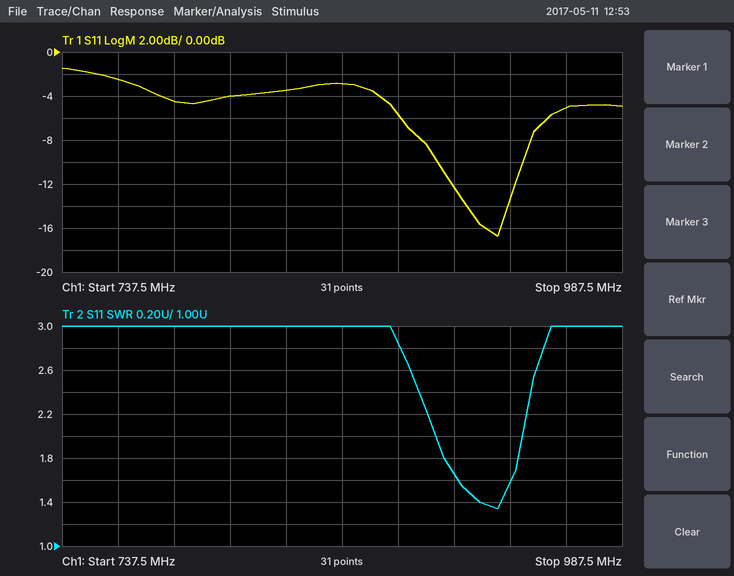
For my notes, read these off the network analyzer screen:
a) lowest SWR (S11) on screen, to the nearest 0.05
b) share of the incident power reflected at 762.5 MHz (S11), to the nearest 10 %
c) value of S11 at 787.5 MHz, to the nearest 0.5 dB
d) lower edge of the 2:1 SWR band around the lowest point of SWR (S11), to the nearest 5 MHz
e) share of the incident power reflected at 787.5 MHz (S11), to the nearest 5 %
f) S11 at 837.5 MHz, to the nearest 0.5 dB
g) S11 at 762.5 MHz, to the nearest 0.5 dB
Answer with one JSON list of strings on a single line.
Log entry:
["1.35", "60 %", "-4.5 dB", "905 MHz", "35 %", "-3.5 dB", "-2.5 dB"]
